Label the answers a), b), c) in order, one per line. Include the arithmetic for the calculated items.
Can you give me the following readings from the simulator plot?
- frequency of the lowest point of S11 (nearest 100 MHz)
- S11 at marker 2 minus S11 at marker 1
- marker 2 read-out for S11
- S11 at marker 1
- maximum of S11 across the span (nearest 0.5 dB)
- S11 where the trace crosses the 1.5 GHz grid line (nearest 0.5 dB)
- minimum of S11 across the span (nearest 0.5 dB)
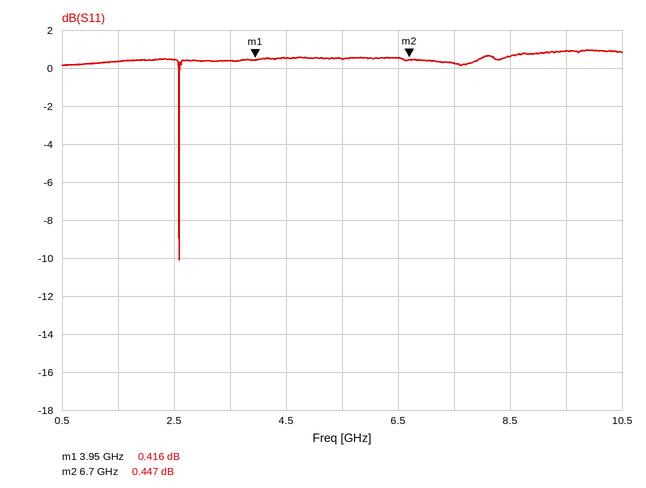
a) 2.6 GHz
b) 0.447 − (0.416) = 0.031 dB
c) 0.447 dB
d) 0.416 dB
e) 1.0 dB
f) 0.5 dB
g) -10.0 dB
